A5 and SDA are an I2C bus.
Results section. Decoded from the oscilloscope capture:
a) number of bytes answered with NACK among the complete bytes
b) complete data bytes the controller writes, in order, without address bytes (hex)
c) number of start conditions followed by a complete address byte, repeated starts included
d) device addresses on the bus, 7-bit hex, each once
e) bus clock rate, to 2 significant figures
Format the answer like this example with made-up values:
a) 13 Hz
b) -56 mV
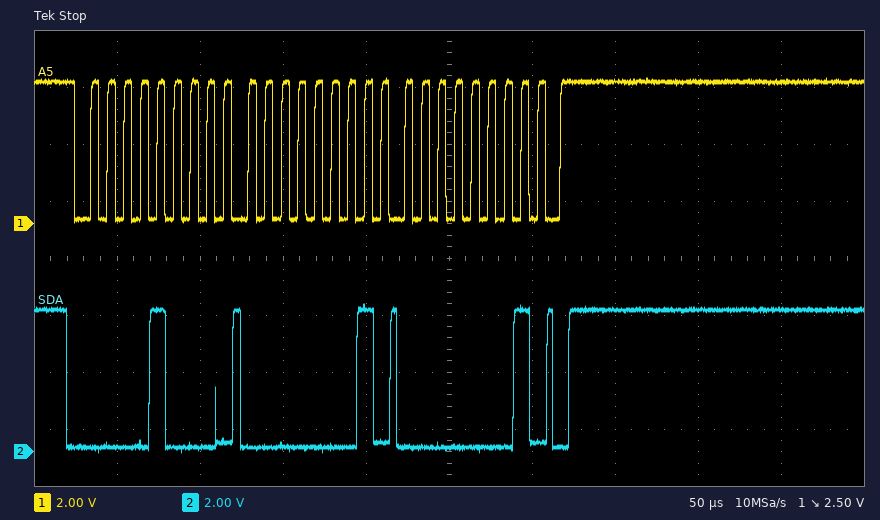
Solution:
a) 0
b) 01 01
c) 1
d) 0x04
e) 100 kHz
